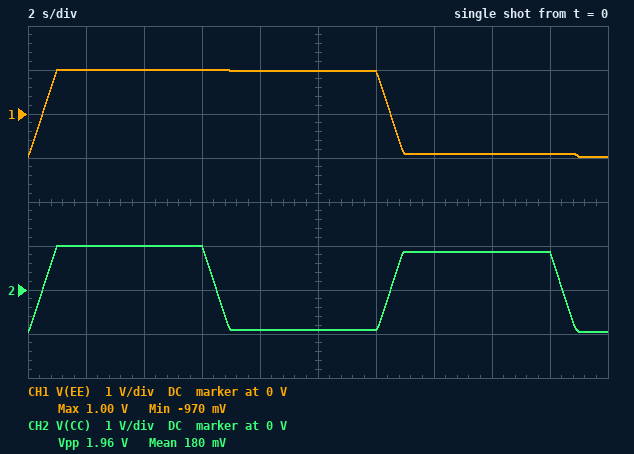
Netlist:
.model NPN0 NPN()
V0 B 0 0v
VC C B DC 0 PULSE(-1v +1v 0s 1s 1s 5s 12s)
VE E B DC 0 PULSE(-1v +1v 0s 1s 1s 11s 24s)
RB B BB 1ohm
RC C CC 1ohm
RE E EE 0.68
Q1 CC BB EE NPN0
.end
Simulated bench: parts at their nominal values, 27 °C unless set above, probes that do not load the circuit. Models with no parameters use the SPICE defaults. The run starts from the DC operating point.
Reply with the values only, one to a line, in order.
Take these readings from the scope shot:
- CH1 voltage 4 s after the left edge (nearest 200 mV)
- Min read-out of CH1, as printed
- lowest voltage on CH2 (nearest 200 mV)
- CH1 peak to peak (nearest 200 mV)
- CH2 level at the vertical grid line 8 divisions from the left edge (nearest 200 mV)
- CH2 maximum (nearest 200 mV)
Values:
1.0 V
-970 mV
-1.0 V
2.0 V
800 mV
1.0 V
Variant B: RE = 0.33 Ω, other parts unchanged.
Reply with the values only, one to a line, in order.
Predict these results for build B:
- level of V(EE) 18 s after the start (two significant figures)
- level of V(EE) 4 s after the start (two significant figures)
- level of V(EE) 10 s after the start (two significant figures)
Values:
-920 mV
1.0 V
990 mV
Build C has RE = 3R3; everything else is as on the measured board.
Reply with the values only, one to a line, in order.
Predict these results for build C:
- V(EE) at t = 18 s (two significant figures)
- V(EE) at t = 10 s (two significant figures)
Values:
-870 mV
860 mV
